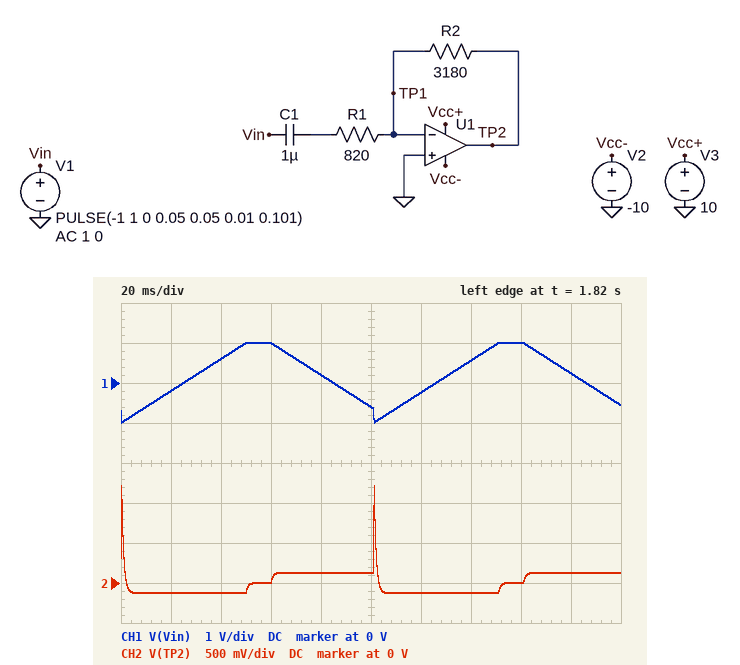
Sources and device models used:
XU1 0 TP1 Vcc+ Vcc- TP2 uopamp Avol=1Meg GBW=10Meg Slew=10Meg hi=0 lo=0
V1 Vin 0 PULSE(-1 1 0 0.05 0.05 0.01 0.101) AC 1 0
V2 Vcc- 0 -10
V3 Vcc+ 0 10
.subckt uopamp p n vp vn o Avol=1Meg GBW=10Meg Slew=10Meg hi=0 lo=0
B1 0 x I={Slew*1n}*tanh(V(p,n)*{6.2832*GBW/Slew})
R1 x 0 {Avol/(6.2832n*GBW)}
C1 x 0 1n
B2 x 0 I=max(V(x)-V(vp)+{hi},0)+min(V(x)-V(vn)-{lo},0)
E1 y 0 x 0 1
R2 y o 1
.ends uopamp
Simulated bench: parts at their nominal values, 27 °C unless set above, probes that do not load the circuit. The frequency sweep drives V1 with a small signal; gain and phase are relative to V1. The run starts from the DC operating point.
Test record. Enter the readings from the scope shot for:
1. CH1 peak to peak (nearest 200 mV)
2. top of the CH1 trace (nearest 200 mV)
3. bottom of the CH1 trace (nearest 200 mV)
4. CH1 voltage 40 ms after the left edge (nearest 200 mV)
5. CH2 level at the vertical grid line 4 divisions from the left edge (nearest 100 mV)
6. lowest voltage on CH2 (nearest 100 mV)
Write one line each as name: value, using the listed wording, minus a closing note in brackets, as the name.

CH1 peak to peak: 2.0 V
top of the CH1 trace: 1.0 V
bottom of the CH1 trace: -1.0 V
CH1 voltage 40 ms after the left edge: 600 mV
CH2 level at the vertical grid line 4 divisions from the left edge: 100 mV
lowest voltage on CH2: -100 mV
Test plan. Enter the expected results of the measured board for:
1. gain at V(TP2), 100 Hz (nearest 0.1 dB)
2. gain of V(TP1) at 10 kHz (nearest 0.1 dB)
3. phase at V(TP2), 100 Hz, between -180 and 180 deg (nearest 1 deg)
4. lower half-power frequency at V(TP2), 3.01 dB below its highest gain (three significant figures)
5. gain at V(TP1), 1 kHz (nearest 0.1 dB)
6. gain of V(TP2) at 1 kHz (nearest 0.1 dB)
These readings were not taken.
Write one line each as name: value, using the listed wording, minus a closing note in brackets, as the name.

gain at V(TP2), 100 Hz: 5.0 dB
gain of V(TP1) at 10 kHz: -48.2 dB
phase at V(TP2), 100 Hz, between -180 and 180 deg: -117 deg
lower half-power frequency at V(TP2), 3.01 dB below its highest gain: 194 Hz
gain at V(TP1), 1 kHz: -68.4 dB
gain of V(TP2) at 1 kHz: 11.6 dB
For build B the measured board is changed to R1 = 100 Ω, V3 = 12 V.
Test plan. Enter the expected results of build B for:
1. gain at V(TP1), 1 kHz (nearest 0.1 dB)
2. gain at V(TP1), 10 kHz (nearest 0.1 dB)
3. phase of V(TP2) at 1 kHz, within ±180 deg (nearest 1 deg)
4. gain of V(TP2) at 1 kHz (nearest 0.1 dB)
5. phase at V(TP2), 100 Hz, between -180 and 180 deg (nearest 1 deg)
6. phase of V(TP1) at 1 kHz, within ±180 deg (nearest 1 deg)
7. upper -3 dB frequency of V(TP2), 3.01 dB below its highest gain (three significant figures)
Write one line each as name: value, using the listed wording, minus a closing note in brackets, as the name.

gain at V(TP1), 1 kHz: -55.4 dB
gain at V(TP1), 10 kHz: -30.0 dB
phase of V(TP2) at 1 kHz, within ±180 deg: -122 deg
gain of V(TP2) at 1 kHz: 24.6 dB
phase at V(TP2), 100 Hz, between -180 and 180 deg: -94 deg
phase of V(TP1) at 1 kHz, within ±180 deg: 147 deg
upper -3 dB frequency of V(TP2), 3.01 dB below its highest gain: 306 kHz
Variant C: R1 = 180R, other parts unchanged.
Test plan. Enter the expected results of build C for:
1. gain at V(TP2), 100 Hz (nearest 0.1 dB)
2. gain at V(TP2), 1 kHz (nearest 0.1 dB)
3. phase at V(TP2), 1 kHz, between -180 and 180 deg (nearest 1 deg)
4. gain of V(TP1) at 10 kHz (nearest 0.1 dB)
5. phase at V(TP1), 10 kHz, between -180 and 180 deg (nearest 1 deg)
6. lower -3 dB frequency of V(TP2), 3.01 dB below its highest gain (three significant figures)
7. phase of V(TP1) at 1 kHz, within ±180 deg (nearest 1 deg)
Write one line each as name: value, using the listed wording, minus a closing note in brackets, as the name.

gain at V(TP2), 100 Hz: 6.0 dB
gain at V(TP2), 1 kHz: 22.4 dB
phase at V(TP2), 1 kHz, between -180 and 180 deg: -139 deg
gain of V(TP1) at 10 kHz: -35.1 dB
phase at V(TP1), 10 kHz, between -180 and 180 deg: 94 deg
lower -3 dB frequency of V(TP2), 3.01 dB below its highest gain: 883 Hz
phase of V(TP1) at 1 kHz, within ±180 deg: 131 deg
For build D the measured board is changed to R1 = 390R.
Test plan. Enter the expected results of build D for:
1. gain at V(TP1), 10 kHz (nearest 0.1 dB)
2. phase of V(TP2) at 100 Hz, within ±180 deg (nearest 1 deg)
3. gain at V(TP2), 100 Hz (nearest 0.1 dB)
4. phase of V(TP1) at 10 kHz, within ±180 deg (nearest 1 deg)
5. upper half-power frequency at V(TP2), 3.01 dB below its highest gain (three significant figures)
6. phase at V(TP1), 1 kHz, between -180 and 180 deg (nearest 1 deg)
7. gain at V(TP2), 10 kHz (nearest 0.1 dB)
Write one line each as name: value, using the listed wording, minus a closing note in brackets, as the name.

gain at V(TP1), 10 kHz: -41.8 dB
phase of V(TP2) at 100 Hz, within ±180 deg: -104 deg
gain at V(TP2), 100 Hz: 5.8 dB
phase of V(TP1) at 10 kHz, within ±180 deg: 92 deg
upper half-power frequency at V(TP2), 3.01 dB below its highest gain: 1.09 MHz
phase at V(TP1), 1 kHz, between -180 and 180 deg: 112 deg
gain at V(TP2), 10 kHz: 18.2 dB
